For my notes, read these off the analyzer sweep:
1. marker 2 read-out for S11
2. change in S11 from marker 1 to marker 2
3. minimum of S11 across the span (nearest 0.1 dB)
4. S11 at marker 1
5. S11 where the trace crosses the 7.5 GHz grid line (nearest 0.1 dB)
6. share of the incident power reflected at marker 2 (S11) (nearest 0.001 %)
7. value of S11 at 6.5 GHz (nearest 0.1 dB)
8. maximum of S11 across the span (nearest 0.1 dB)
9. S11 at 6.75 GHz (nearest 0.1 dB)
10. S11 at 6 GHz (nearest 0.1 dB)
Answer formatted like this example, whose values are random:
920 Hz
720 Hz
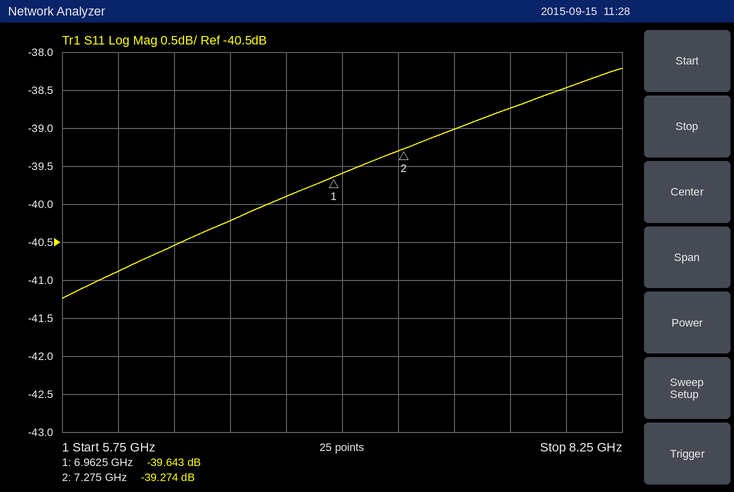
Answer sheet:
-39.274 dB
0.369 dB
-41.2 dB
-39.643 dB
-39.0 dB
0.012 %
-40.2 dB
-38.2 dB
-39.9 dB
-40.9 dB
